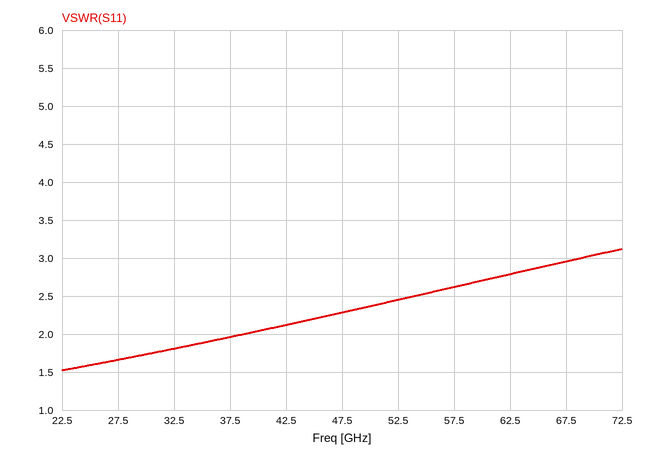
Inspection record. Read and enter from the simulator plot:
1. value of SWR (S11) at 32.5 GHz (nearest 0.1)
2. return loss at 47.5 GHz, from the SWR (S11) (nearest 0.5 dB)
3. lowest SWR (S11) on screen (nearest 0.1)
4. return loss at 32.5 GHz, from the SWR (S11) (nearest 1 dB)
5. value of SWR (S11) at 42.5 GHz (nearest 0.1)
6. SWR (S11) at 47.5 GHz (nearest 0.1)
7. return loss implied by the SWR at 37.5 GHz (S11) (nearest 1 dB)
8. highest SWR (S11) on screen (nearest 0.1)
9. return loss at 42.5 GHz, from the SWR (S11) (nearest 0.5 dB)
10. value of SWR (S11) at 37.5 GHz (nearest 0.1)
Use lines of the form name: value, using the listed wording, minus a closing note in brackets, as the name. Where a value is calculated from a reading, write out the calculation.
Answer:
value of SWR (S11) at 32.5 GHz: 1.8
return loss at 47.5 GHz, from the SWR (S11): −20 log10((2.3 − 1)/(2.3 + 1)) ≈ 8.09 dB, so 8.0 dB to the nearest 0.5 dB
lowest SWR (S11) on screen: 1.5
return loss at 32.5 GHz, from the SWR (S11): −20 log10((1.8 − 1)/(1.8 + 1)) ≈ 11 dB
value of SWR (S11) at 42.5 GHz: 2.1
SWR (S11) at 47.5 GHz: 2.3
return loss implied by the SWR at 37.5 GHz (S11): −20 log10((2 − 1)/(2 + 1)) ≈ 10 dB
highest SWR (S11) on screen: 3.1
return loss at 42.5 GHz, from the SWR (S11): −20 log10((2.1 − 1)/(2.1 + 1)) ≈ 9.0 dB
value of SWR (S11) at 37.5 GHz: 2.0
